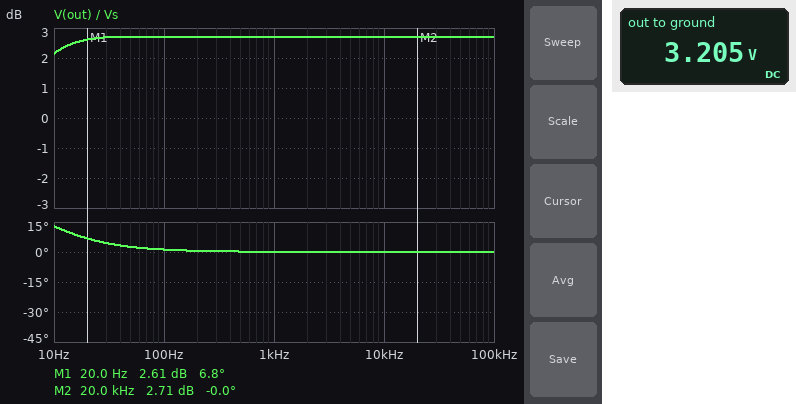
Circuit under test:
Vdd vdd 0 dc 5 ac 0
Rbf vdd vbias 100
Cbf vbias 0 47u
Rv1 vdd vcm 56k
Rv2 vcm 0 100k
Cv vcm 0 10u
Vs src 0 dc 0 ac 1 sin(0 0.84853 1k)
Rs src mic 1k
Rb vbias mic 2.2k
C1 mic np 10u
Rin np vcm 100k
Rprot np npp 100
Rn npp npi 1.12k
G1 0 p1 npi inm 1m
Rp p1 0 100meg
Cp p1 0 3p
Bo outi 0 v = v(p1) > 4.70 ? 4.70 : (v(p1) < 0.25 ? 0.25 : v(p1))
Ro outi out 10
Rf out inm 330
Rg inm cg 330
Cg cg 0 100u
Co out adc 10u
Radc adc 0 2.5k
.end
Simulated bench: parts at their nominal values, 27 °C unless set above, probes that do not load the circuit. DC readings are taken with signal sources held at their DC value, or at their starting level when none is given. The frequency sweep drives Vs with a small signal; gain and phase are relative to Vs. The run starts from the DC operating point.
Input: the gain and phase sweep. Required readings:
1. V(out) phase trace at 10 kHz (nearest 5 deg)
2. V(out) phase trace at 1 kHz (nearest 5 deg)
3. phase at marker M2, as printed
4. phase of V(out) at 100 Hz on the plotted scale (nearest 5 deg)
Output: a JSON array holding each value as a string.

["0 deg", "0 deg", "-0.0 deg", "0 deg"]
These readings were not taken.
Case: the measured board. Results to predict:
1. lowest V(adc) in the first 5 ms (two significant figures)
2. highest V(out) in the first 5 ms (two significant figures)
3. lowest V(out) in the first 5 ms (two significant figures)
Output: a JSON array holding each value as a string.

["-1.2 V", "4.4 V", "2.0 V"]
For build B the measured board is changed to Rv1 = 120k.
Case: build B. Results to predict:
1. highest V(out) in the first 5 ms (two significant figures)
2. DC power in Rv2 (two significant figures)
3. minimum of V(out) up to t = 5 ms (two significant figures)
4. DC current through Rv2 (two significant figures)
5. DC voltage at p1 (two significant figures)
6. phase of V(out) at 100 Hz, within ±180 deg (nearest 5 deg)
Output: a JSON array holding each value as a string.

["3.4 V", "52 µW", "1.1 V", "23 µA", "2.3 V", "0 deg"]
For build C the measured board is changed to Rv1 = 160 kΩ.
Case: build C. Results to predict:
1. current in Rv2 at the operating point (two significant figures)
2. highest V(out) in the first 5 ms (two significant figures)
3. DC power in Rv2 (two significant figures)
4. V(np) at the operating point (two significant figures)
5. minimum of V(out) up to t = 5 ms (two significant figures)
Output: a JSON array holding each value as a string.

["19 µA", "3.1 V", "37 µW", "1.9 V", "760 mV"]
